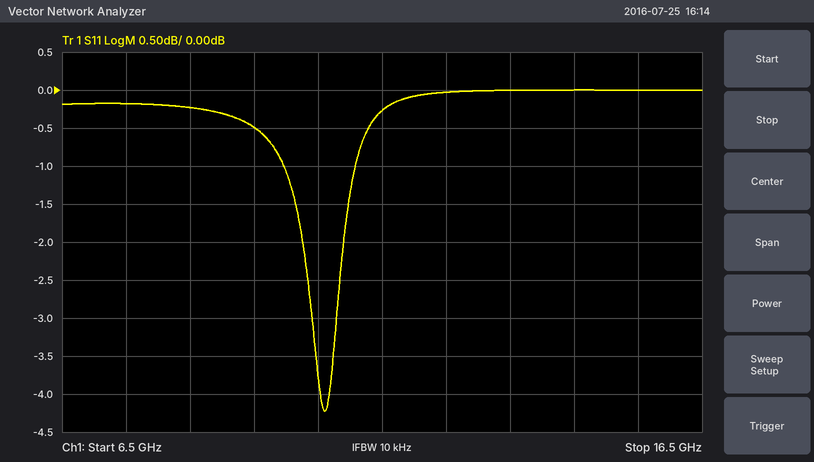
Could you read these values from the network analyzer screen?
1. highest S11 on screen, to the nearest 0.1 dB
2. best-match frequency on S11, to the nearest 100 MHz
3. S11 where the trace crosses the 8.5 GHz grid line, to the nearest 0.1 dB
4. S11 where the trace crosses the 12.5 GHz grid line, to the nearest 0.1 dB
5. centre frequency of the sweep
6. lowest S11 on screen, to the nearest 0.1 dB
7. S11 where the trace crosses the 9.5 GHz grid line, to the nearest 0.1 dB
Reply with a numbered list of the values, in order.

1. 0.0 dB
2. 10.6 GHz
3. -0.2 dB
4. 0.0 dB
5. 11.5 GHz
6. -4.2 dB
7. -0.5 dB
